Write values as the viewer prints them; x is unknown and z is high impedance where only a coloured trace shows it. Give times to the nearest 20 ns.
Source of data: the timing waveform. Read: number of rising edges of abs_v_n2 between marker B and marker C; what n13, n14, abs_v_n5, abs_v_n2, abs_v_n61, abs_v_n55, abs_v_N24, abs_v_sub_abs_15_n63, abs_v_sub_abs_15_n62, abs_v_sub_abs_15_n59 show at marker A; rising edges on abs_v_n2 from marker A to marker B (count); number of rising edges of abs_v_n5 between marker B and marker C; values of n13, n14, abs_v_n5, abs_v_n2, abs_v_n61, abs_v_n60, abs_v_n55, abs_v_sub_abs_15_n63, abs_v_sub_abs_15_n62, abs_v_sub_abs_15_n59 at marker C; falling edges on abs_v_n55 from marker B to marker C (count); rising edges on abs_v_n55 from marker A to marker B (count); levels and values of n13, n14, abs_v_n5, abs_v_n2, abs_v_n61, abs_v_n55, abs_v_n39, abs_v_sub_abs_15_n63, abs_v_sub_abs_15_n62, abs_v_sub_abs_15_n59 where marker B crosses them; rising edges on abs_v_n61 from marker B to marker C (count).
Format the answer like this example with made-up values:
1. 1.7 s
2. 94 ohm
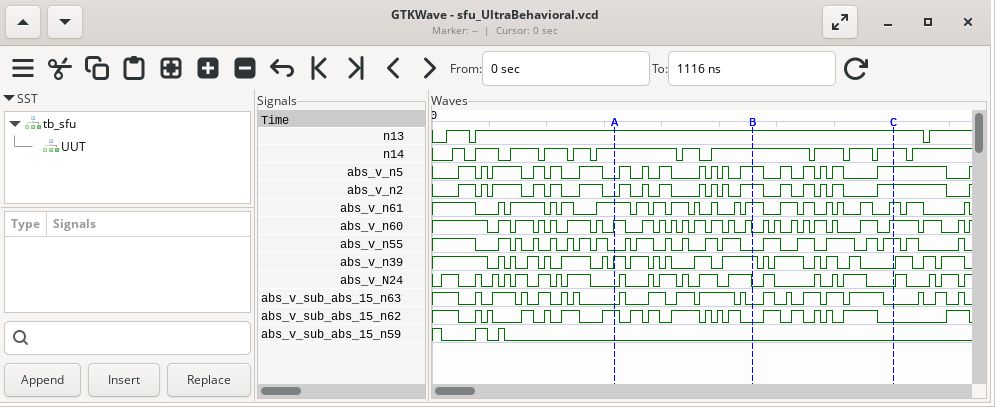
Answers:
1. 5
2. n13=1, n14=1, abs_v_n5=0, abs_v_n2=0, abs_v_n61=1, abs_v_n55=0, abs_v_N24=0, abs_v_sub_abs_15_n63=0, abs_v_sub_abs_15_n62=1, abs_v_sub_abs_15_n59=0
3. 7
4. 5
5. n13=1, n14=1, abs_v_n5=1, abs_v_n2=1, abs_v_n61=1, abs_v_n60=1, abs_v_n55=1, abs_v_sub_abs_15_n63=0, abs_v_sub_abs_15_n62=0, abs_v_sub_abs_15_n59=0
6. 4
7. 6
8. n13=1, n14=1, abs_v_n5=1, abs_v_n2=1, abs_v_n61=1, abs_v_n55=0, abs_v_n39=1, abs_v_sub_abs_15_n63=0, abs_v_sub_abs_15_n62=0, abs_v_sub_abs_15_n59=0
9. 6
